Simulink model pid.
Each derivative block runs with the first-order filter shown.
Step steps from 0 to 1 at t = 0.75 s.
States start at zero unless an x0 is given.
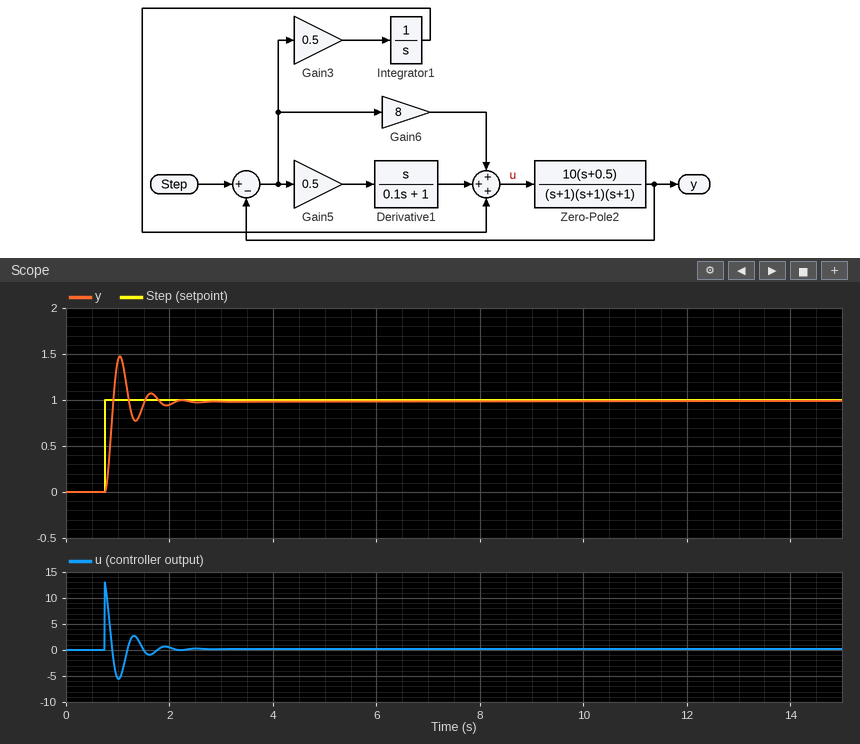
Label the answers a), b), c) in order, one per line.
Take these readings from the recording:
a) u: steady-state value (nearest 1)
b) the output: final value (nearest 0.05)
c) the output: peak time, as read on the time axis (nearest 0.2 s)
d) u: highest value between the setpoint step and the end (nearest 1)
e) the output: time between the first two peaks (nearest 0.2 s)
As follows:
a) 0
b) 1.00
c) 1.0 s
d) 13
e) 0.6 s
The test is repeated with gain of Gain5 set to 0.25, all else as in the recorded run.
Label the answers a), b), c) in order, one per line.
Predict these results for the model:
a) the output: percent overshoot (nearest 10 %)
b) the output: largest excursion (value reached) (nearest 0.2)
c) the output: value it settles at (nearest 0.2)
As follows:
a) 50 %
b) 1.6
c) 1.0
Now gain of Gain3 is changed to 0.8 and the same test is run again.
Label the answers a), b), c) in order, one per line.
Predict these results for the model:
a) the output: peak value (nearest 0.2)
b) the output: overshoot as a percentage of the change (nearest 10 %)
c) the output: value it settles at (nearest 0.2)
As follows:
a) 1.4
b) 50 %
c) 1.0
